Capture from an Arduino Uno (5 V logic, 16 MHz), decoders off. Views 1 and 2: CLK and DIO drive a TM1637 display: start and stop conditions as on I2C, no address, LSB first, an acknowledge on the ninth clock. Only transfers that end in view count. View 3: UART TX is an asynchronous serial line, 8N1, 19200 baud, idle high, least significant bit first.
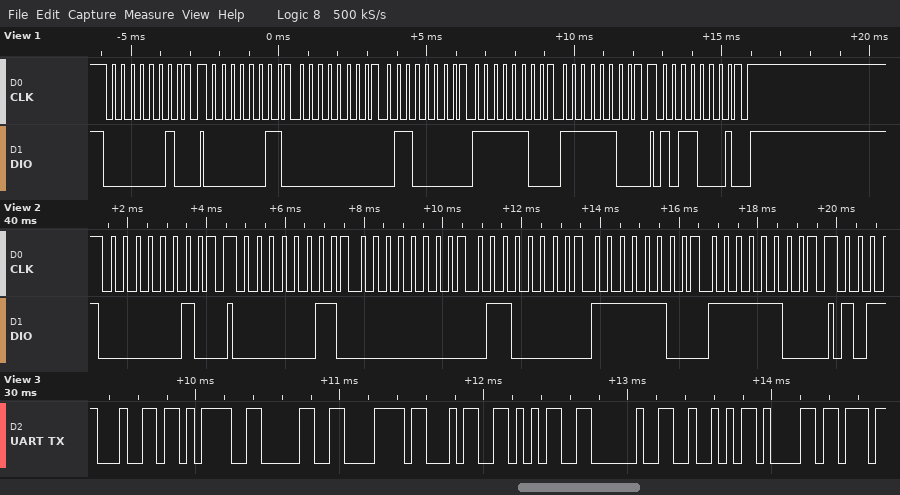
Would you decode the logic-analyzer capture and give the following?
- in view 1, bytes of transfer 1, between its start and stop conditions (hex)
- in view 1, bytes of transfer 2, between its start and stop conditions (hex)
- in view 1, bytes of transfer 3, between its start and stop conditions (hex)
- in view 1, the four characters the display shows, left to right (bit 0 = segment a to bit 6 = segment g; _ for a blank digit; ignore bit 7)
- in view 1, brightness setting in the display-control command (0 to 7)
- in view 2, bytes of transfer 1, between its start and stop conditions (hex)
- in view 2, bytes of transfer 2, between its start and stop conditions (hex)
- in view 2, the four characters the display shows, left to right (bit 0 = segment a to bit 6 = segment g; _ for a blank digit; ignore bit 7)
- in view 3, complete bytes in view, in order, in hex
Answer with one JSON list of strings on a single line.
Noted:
["40", "C0 00 06 3F 3F", "8D", "_100", "5", "40", "C0 00 06 3F 3F", "_100", "0x64 0x3D 0x30 0x78 0x34 0x35 0x20 0x52 0x61"]
